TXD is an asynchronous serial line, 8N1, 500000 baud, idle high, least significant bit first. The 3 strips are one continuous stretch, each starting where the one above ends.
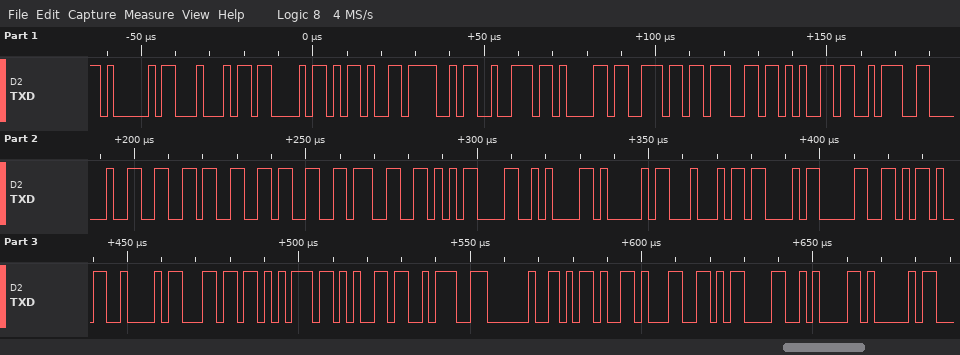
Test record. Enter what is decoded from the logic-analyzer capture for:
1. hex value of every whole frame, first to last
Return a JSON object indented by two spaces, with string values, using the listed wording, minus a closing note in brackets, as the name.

{
  "hex value of every whole frame, first to last": "41 44 43 2D 4F 72 61 6E 67 65 3A 20 66 66 66 66 0D 0A 41 44 43 30 2D 42 6C 75 65 3A 20 2D 31 0D 0A 41"
}
